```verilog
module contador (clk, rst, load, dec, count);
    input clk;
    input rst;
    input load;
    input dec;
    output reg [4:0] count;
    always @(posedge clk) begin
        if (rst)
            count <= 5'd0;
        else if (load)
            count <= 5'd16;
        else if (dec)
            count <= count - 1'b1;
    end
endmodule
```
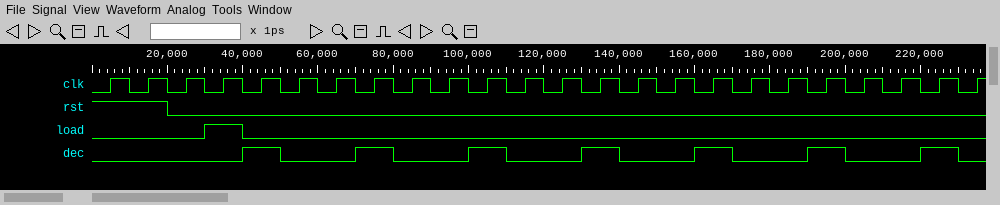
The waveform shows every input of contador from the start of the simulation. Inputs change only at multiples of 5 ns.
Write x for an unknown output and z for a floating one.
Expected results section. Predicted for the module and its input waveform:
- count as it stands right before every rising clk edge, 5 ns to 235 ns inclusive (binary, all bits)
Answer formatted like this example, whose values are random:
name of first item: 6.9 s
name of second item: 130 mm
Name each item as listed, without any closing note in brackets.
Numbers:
count as it stands right before every rising clk edge, 5 ns to 235 ns inclusive: x, 00000, 00000, 00000, 10000, 01111, 01111, 01111, 01110, 01110, 01110, 01101, 01101, 01101, 01100, 01100, 01100, 01011, 01011, 01011, 01010, 01010, 01010, 01001
